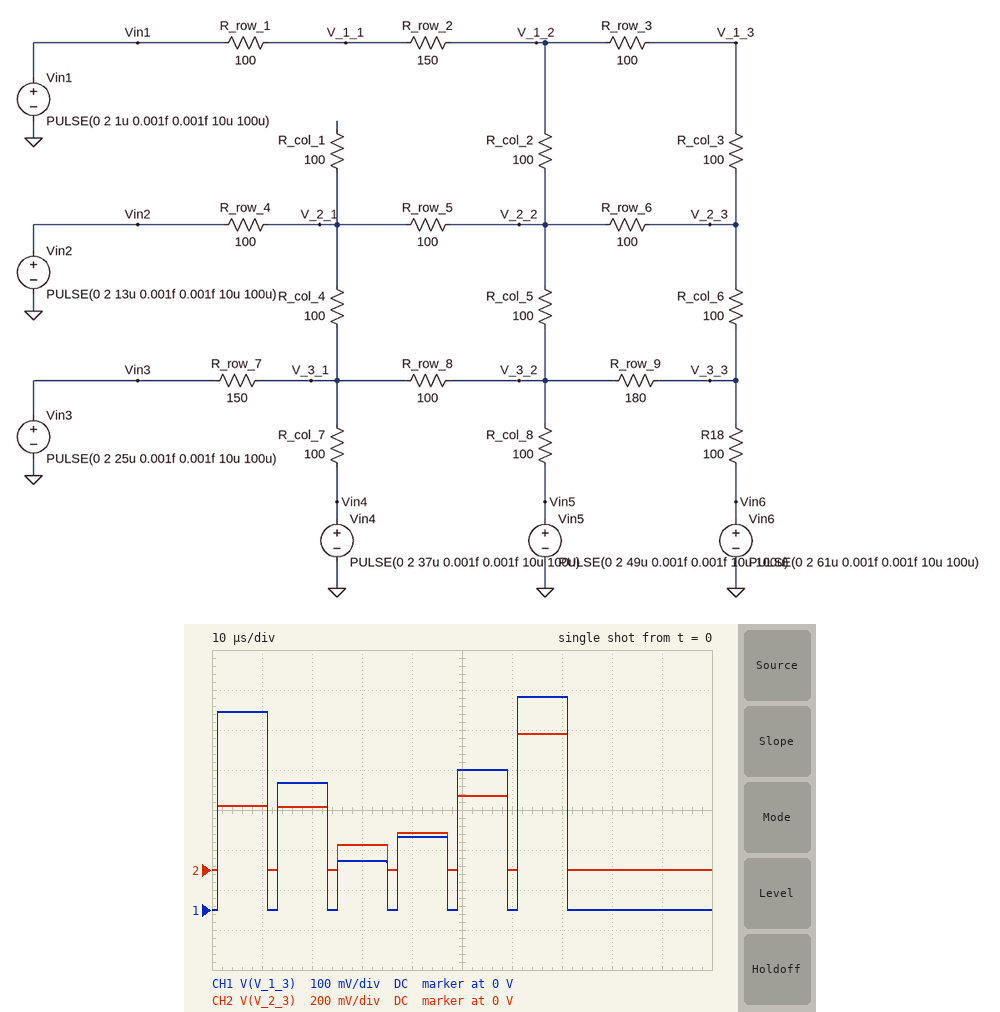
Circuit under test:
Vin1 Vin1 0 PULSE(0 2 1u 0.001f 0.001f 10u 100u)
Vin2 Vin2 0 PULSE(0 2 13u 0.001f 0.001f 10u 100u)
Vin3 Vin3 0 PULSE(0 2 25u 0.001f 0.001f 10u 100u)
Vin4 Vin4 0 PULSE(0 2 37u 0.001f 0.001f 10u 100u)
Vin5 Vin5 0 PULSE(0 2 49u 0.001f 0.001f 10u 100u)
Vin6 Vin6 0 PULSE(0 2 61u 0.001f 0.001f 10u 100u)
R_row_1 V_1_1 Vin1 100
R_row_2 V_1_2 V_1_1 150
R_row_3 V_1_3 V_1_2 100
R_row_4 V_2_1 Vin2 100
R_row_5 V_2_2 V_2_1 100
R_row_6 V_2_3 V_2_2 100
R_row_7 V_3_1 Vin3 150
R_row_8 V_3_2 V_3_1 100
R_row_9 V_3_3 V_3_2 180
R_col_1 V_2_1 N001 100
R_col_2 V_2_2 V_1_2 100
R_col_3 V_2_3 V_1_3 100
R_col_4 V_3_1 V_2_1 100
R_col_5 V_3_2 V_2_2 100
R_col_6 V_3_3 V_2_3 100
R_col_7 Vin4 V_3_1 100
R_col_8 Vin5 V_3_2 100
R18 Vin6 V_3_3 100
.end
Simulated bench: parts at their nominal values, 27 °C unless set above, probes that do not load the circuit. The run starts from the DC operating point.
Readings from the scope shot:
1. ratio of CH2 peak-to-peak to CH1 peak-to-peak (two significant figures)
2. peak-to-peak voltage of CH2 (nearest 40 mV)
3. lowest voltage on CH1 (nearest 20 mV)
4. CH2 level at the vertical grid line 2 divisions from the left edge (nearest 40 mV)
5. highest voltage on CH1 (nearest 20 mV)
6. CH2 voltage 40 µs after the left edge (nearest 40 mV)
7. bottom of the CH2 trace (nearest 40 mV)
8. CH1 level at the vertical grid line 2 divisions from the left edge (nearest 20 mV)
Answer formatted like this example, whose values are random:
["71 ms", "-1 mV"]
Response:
["1.3", "680 mV", "0 V", "320 mV", "540 mV", "200 mV", "0 V", "320 mV"]
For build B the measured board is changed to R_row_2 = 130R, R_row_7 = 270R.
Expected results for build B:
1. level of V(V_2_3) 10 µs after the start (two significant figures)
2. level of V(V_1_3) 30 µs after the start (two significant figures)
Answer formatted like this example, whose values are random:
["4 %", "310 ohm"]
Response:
["340 mV", "74 mV"]
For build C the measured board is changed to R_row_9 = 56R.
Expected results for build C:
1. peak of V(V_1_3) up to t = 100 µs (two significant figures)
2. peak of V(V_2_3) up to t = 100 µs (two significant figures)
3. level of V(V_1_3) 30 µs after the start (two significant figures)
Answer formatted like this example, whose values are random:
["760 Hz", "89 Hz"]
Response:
["490 mV", "600 mV", "130 mV"]
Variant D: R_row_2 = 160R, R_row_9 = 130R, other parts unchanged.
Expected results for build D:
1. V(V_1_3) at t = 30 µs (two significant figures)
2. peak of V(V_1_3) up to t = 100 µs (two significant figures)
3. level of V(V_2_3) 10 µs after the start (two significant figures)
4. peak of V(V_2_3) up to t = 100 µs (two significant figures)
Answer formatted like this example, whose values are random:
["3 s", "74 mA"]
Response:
["120 mV", "520 mV", "310 mV", "660 mV"]
